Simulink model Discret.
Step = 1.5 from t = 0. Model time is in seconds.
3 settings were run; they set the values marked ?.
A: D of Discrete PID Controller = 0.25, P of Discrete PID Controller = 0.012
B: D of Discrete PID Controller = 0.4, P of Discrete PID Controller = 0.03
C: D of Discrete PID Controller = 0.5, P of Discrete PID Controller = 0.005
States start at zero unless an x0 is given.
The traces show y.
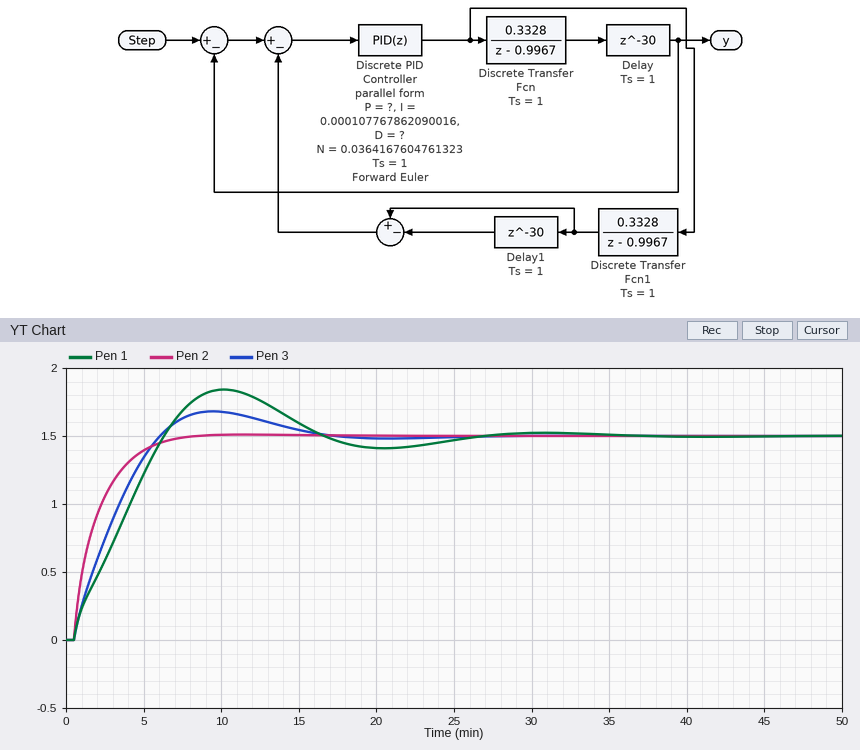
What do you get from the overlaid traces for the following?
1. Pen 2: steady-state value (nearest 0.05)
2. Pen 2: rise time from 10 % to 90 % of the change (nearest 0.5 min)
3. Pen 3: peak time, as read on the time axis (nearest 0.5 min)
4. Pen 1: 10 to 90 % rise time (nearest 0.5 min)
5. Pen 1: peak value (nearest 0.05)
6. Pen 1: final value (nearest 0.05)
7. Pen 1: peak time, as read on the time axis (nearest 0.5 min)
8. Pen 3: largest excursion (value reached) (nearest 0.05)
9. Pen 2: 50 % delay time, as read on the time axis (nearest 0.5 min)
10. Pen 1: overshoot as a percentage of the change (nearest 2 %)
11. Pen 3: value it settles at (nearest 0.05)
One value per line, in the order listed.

1.50
4.0 min
9.5 min
5.0 min
1.85
1.50
10.0 min
1.70
1.5 min
22 %
1.50
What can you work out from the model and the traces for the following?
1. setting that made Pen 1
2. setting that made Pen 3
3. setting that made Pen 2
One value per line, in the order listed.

C
A
B
